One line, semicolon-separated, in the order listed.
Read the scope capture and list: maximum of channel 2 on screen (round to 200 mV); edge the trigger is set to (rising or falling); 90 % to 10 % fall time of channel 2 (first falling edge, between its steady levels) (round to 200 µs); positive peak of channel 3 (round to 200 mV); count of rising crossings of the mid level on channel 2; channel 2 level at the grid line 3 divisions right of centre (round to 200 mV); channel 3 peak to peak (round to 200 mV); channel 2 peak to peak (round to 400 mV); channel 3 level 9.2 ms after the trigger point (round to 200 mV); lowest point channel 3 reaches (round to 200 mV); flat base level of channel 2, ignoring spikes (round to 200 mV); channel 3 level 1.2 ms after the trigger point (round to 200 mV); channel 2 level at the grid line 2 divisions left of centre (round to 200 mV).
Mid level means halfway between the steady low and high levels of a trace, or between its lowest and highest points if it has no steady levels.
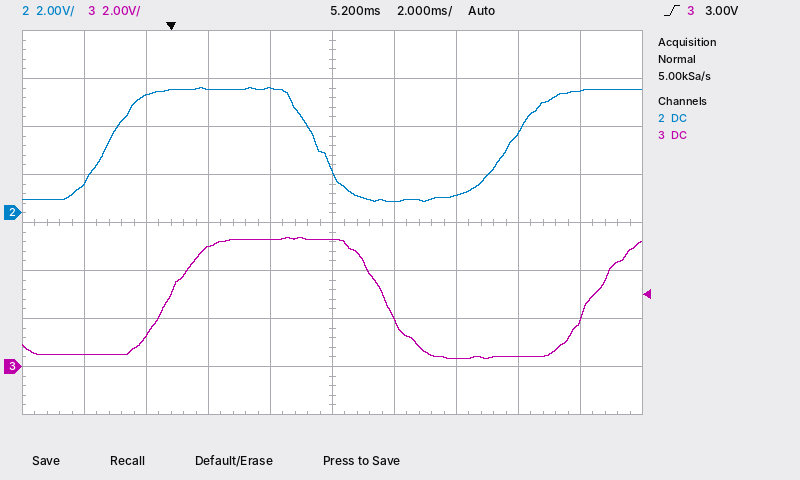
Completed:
5.2 V; rising; 1.8 ms; 5.4 V; 2; 3.4 V; 5.0 V; 4.8 V; 400 mV; 400 mV; 600 mV; 5.0 V; 5.2 V
